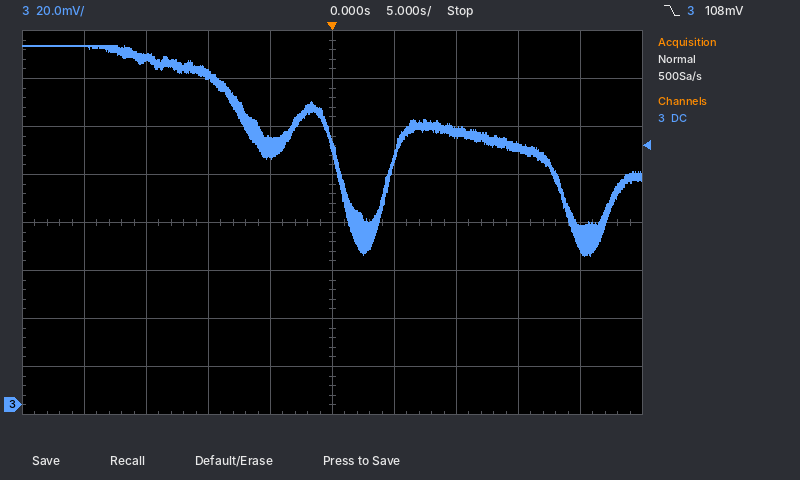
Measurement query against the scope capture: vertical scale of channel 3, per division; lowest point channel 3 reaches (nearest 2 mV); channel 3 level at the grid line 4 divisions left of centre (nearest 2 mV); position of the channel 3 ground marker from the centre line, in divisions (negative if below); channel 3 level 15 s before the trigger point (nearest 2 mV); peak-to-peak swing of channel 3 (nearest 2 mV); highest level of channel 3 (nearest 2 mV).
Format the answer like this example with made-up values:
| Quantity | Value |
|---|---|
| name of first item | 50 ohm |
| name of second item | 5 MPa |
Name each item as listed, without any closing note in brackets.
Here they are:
| Quantity | Value |
|---|---|
| vertical scale of channel 3, per division | 20 mV |
| lowest point channel 3 reaches | 62 mV |
| channel 3 level at the grid line 4 divisions left of centre | 150 mV |
| position of the channel 3 ground marker from the centre line, in divisions | -3.8 div |
| channel 3 level 15 s before the trigger point | 144 mV |
| peak-to-peak swing of channel 3 | 88 mV |
| highest level of channel 3 | 150 mV |
